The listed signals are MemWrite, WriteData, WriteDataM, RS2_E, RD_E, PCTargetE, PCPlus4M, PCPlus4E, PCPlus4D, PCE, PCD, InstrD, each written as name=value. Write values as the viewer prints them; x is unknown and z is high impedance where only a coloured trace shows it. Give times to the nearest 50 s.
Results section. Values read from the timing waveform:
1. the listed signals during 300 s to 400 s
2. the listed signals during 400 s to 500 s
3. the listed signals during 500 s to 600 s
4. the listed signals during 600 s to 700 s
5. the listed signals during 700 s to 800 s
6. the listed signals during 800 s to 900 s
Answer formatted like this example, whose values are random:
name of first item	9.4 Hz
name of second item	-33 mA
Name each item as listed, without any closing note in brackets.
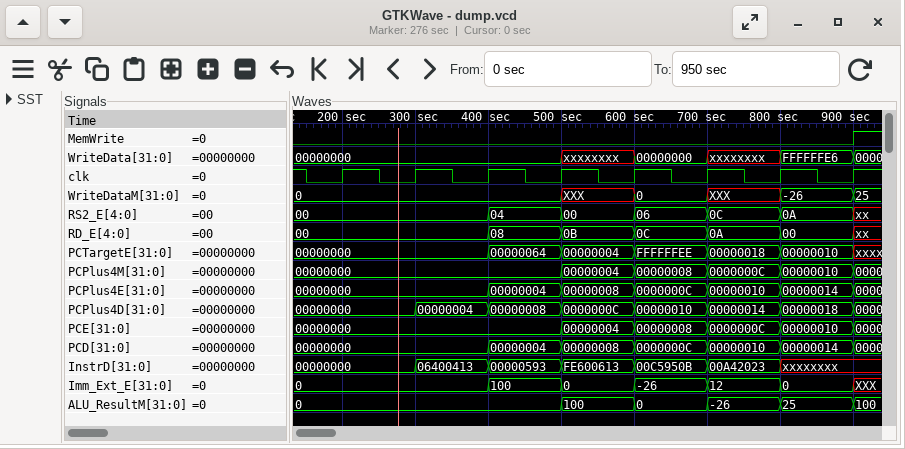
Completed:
the listed signals during 300 s to 400 s	MemWrite=0, WriteData=00000000, WriteDataM=0, RS2_E=00, RD_E=00, PCTargetE=00000000, PCPlus4M=00000000, PCPlus4E=00000000, PCPlus4D=00000004, PCE=00000000, PCD=00000000, InstrD=06400413
the listed signals during 400 s to 500 s	MemWrite=0, WriteData=00000000, WriteDataM=0, RS2_E=04, RD_E=08, PCTargetE=00000064, PCPlus4M=00000000, PCPlus4E=00000004, PCPlus4D=00000008, PCE=00000000, PCD=00000004, InstrD=00000593
the listed signals during 500 s to 600 s	MemWrite=0, WriteData=xxxxxxxx, WriteDataM=XXX, RS2_E=00, RD_E=0B, PCTargetE=00000004, PCPlus4M=00000004, PCPlus4E=00000008, PCPlus4D=0000000C, PCE=00000004, PCD=00000008, InstrD=FE600613
the listed signals during 600 s to 700 s	MemWrite=0, WriteData=00000000, WriteDataM=0, RS2_E=06, RD_E=0C, PCTargetE=FFFFFFEE, PCPlus4M=00000008, PCPlus4E=0000000C, PCPlus4D=00000010, PCE=00000008, PCD=0000000C, InstrD=00C5950B
the listed signals during 700 s to 800 s	MemWrite=0, WriteData=xxxxxxxx, WriteDataM=XXX, RS2_E=0C, RD_E=0A, PCTargetE=00000018, PCPlus4M=0000000C, PCPlus4E=00000010, PCPlus4D=00000014, PCE=0000000C, PCD=00000010, InstrD=00A42023
the listed signals during 800 s to 900 s	MemWrite=0, WriteData=FFFFFFE6, WriteDataM=-26, RS2_E=0A, RD_E=00, PCTargetE=00000010, PCPlus4M=00000010, PCPlus4E=00000014, PCPlus4D=00000018, PCE=00000010, PCD=00000014, InstrD=xxxxxxxx
